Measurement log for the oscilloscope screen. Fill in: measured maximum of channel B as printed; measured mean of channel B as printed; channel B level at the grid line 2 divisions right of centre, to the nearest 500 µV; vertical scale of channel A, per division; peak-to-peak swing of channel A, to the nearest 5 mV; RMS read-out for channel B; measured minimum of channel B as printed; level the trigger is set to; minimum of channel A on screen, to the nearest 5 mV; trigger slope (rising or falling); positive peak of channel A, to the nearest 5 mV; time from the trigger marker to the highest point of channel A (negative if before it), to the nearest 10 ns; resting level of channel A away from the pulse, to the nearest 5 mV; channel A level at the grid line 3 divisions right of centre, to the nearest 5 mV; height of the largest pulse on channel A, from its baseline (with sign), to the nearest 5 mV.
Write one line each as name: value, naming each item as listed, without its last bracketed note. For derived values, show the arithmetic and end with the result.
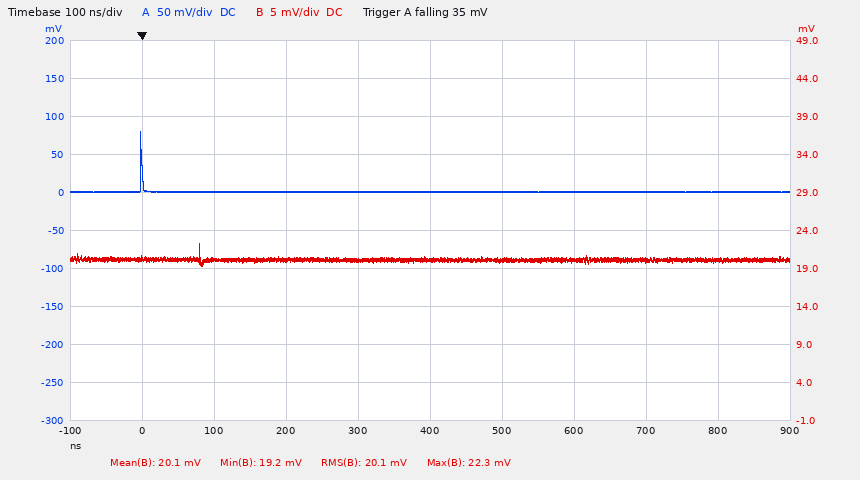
measured maximum of channel B as printed: 22.3 mV
measured mean of channel B as printed: 20.1 mV
channel B level at the grid line 2 divisions right of centre, to the nearest 500 µV: 20.0 mV
vertical scale of channel A, per division: 50 mV
peak-to-peak swing of channel A, to the nearest 5 mV: 80 mV − (0 mV) = 80 mV
RMS read-out for channel B: 20.1 mV
measured minimum of channel B as printed: 19.2 mV
level the trigger is set to: 35 mV
minimum of channel A on screen, to the nearest 5 mV: 0 mV
trigger slope: falling
positive peak of channel A, to the nearest 5 mV: 80 mV
time from the trigger marker to the highest point of channel A (negative if before it), to the nearest 10 ns: 0 ns
resting level of channel A away from the pulse, to the nearest 5 mV: 0 mV
channel A level at the grid line 3 divisions right of centre, to the nearest 5 mV: 0 mV
height of the largest pulse on channel A, from its baseline (with sign), to the nearest 5 mV: 80 mV − (0 mV) = +80 mV
